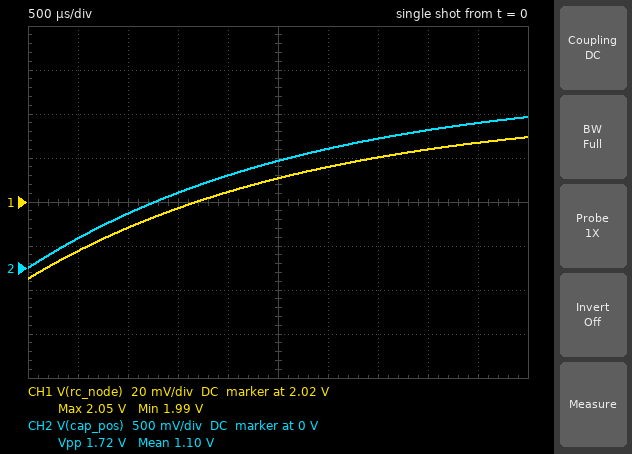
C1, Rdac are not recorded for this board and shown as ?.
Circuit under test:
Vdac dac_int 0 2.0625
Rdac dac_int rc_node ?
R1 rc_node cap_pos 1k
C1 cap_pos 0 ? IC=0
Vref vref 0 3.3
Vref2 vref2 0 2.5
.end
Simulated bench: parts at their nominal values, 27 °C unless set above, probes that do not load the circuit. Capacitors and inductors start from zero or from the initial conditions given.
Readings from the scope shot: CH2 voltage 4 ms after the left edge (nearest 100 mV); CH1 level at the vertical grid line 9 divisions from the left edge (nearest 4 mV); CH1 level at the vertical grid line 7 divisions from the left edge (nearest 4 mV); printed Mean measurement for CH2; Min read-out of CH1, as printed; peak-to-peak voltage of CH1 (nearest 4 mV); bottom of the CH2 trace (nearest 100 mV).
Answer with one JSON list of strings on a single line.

["1.6 V", "2.048 V", "2.040 V", "1.10 V", "1.99 V", "64 mV", "0 V"]
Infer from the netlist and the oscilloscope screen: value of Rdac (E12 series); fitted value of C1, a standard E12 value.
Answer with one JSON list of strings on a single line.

["39 Ω", "2.7 µF"]
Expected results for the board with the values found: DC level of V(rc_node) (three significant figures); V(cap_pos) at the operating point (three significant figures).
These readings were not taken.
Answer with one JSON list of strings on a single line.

["2.06 V", "2.06 V"]
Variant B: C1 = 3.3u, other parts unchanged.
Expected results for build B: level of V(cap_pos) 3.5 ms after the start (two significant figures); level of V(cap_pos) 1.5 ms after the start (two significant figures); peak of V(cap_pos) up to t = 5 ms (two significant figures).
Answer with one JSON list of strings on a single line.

["1.3 V", "730 mV", "1.6 V"]
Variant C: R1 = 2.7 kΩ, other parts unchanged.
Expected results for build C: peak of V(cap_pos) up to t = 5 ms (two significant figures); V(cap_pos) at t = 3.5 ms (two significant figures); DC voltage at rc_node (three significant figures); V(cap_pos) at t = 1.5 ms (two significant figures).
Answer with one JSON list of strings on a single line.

["1.0 V", "780 mV", "2.06 V", "380 mV"]
